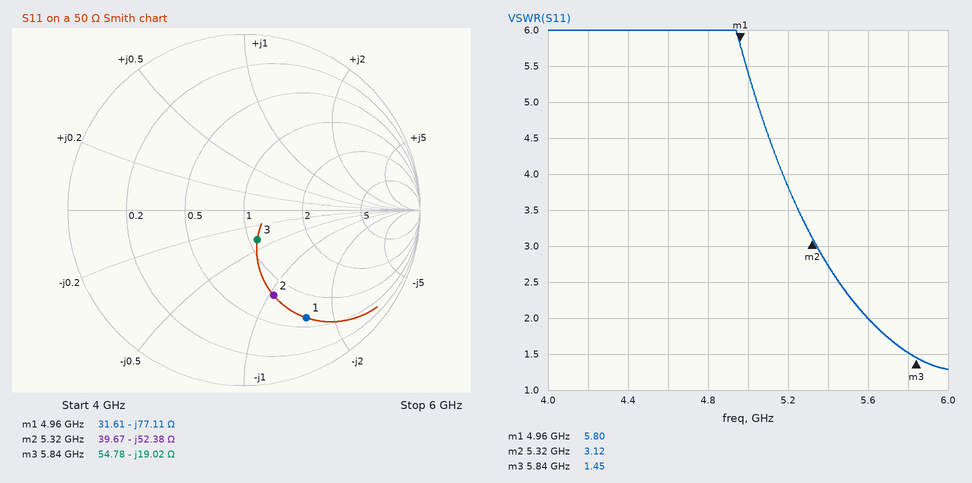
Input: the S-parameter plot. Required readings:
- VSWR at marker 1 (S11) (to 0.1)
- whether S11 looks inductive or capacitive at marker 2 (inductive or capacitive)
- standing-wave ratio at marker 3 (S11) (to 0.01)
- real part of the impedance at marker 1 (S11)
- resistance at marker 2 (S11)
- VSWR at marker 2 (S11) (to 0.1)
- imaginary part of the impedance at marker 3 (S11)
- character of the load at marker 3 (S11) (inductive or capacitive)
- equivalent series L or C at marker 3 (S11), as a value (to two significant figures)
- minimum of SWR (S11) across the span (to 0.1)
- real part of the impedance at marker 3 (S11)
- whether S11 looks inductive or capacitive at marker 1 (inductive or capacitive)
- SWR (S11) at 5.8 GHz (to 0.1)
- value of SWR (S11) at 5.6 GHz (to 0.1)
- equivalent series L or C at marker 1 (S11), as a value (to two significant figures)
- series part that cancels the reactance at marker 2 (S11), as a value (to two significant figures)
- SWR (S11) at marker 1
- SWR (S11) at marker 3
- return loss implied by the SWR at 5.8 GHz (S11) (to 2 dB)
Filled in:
5.8
capacitive
1.45
31.61 Ω
39.67 Ω
3.1
-19.02 Ω
capacitive
1.4 pF
1.3
54.78 Ω
capacitive
1.5
2.0
420 fF
1.6 nH
5.80
1.45
14 dB
